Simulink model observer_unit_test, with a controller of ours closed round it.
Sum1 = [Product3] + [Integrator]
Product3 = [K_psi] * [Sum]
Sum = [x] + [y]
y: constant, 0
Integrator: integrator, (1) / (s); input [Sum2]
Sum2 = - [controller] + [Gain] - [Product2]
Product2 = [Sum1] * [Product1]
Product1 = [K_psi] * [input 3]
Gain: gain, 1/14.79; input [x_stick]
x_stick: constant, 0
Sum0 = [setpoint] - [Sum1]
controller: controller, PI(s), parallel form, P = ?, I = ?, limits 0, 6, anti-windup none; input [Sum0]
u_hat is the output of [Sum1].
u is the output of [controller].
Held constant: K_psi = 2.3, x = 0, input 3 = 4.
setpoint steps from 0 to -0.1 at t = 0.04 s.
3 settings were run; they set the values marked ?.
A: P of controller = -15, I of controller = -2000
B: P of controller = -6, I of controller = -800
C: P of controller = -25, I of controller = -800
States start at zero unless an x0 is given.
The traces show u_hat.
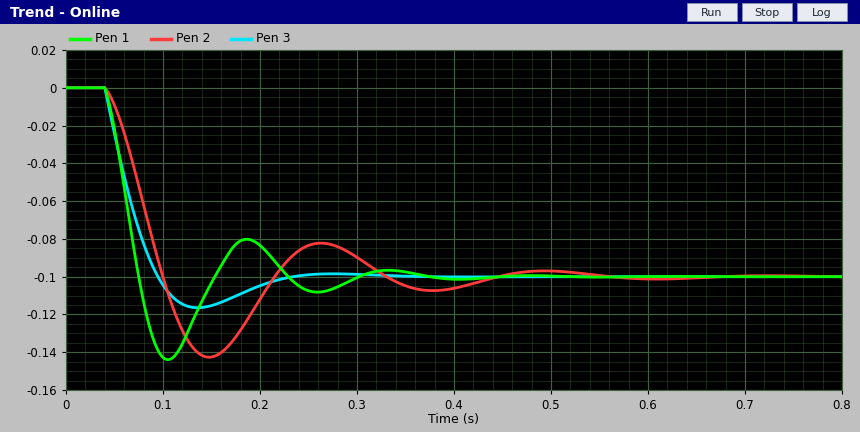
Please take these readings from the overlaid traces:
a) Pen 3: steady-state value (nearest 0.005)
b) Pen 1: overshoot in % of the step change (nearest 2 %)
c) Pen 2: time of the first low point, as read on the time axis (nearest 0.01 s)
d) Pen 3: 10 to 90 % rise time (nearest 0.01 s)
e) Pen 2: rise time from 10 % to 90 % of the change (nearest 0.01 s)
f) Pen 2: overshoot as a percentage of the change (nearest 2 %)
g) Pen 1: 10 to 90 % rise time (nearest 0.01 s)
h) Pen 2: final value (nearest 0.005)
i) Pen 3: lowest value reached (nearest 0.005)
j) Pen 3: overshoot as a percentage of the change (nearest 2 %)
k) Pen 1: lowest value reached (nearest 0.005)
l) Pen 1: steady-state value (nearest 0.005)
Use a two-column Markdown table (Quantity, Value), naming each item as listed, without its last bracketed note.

| Quantity | Value |
|---|---|
| Pen 3: steady-state value | -0.100 |
| Pen 1: overshoot in % of the step change | 44 % |
| Pen 2: time of the first low point, as read on the time axis | 0.15 s |
| Pen 3: 10 to 90 % rise time | 0.04 s |
| Pen 2: rise time from 10 % to 90 % of the change | 0.04 s |
| Pen 2: overshoot as a percentage of the change | 42 % |
| Pen 1: 10 to 90 % rise time | 0.03 s |
| Pen 2: final value | -0.100 |
| Pen 3: lowest value reached | -0.115 |
| Pen 3: overshoot as a percentage of the change | 16 % |
| Pen 1: lowest value reached | -0.145 |
| Pen 1: steady-state value | -0.100 |
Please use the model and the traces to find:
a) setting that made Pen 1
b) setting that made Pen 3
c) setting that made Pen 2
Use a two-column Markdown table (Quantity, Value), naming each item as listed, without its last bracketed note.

| Quantity | Value |
|---|---|
| setting that made Pen 1 | A |
| setting that made Pen 3 | C |
| setting that made Pen 2 | B |
